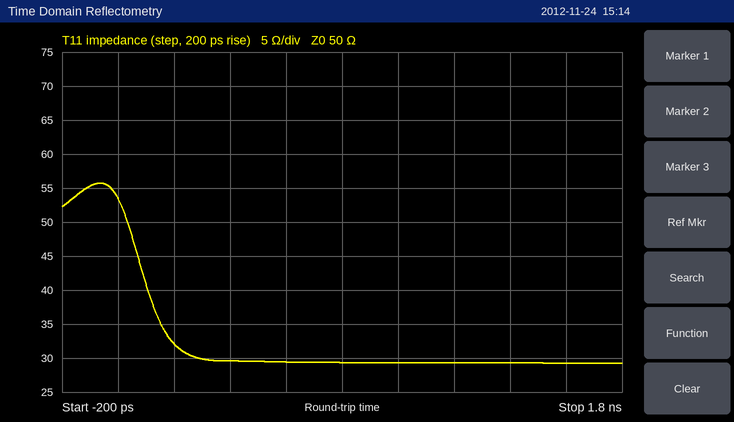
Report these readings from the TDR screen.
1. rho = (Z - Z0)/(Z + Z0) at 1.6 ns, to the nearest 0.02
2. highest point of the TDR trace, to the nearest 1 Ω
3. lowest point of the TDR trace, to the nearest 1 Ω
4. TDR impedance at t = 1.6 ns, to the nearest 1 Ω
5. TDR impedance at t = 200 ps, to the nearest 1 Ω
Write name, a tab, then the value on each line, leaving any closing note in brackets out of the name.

rho = (Z - Z0)/(Z + Z0) at 1.6 ns, to the nearest 0.02	-0.26
highest point of the TDR trace, to the nearest 1 Ω	56 Ω
lowest point of the TDR trace, to the nearest 1 Ω	29 Ω
TDR impedance at t = 1.6 ns, to the nearest 1 Ω	29 Ω
TDR impedance at t = 200 ps, to the nearest 1 Ω	32 Ω
